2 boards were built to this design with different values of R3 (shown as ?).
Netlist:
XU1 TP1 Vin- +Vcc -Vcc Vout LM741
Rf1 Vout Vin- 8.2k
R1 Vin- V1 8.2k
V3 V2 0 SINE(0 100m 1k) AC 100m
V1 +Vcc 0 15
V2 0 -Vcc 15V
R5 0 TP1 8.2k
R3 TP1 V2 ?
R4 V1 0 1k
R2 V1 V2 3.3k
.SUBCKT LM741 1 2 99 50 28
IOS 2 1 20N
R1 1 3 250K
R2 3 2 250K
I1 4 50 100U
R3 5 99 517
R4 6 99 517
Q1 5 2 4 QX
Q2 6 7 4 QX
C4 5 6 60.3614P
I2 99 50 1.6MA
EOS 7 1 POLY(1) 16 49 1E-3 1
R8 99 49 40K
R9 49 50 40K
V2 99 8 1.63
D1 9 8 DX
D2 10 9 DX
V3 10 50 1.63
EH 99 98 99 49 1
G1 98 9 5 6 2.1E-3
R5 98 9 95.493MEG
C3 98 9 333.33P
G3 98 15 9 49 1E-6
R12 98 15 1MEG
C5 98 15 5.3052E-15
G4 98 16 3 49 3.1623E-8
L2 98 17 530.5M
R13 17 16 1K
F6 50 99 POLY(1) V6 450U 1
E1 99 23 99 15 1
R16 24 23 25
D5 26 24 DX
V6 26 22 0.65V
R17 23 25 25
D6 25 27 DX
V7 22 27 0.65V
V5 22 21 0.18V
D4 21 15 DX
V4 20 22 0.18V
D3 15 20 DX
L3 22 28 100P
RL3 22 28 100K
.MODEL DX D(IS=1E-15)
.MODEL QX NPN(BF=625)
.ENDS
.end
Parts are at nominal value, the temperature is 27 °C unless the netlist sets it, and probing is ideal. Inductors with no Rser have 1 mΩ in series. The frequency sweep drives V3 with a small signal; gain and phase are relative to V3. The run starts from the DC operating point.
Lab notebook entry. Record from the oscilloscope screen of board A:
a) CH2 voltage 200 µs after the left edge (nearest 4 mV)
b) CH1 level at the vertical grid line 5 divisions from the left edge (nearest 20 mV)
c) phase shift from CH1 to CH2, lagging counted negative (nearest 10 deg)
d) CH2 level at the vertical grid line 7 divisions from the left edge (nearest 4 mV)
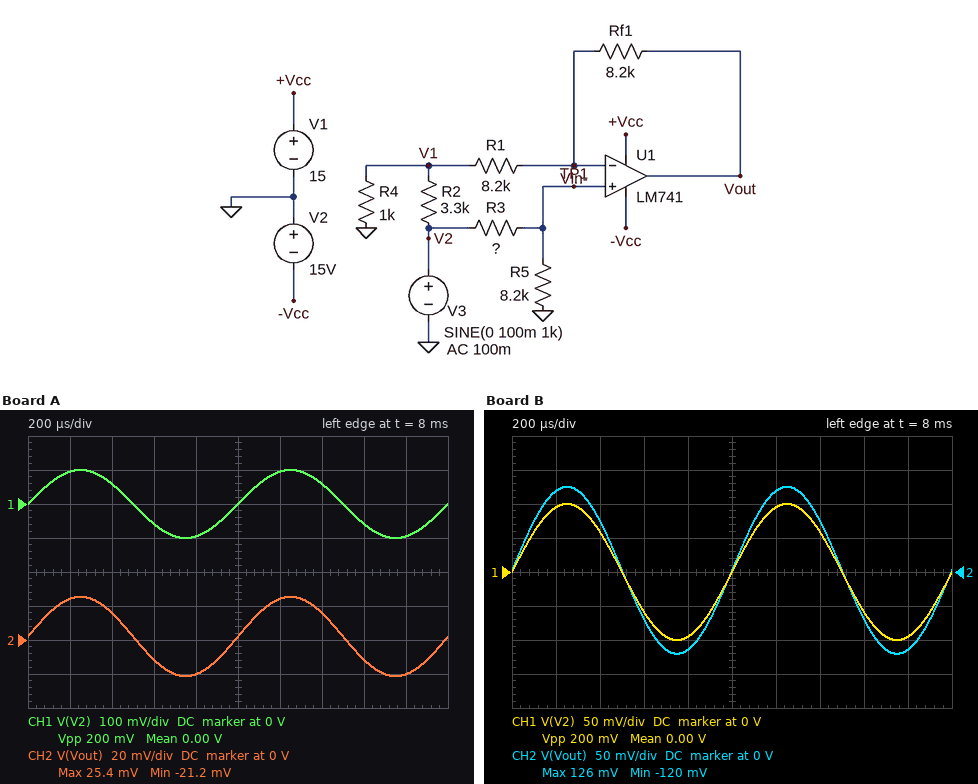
24 mV
0 V
0 deg
16 mV
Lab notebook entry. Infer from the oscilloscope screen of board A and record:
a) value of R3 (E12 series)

27 kΩ
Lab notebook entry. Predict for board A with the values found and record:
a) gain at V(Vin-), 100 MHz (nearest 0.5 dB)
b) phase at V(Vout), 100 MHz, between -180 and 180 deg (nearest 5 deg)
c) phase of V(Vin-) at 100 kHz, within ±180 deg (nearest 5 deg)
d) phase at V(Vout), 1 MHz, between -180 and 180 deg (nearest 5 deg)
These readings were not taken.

-19.0 dB
5 deg
-5 deg
-75 deg
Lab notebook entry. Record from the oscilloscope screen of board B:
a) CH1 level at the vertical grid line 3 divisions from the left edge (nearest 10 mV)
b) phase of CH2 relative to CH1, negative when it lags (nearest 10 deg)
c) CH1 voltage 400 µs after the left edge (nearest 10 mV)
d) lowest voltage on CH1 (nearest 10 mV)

-60 mV
0 deg
60 mV
-100 mV
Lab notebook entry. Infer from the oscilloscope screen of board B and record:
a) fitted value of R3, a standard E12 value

2.7 kΩ
